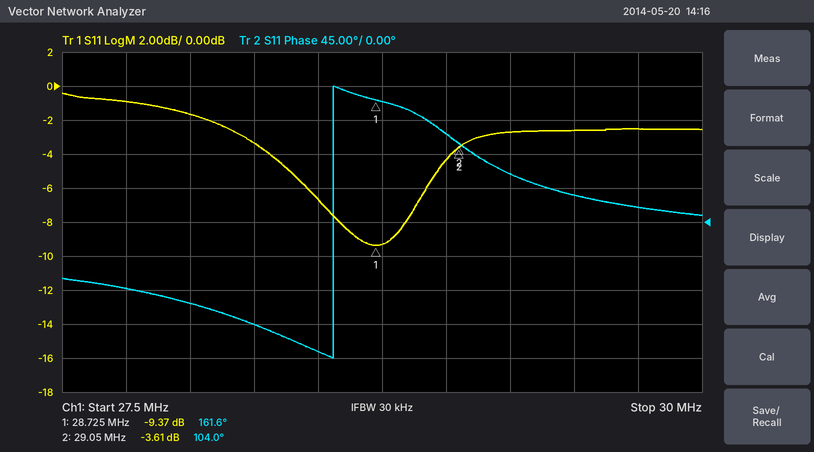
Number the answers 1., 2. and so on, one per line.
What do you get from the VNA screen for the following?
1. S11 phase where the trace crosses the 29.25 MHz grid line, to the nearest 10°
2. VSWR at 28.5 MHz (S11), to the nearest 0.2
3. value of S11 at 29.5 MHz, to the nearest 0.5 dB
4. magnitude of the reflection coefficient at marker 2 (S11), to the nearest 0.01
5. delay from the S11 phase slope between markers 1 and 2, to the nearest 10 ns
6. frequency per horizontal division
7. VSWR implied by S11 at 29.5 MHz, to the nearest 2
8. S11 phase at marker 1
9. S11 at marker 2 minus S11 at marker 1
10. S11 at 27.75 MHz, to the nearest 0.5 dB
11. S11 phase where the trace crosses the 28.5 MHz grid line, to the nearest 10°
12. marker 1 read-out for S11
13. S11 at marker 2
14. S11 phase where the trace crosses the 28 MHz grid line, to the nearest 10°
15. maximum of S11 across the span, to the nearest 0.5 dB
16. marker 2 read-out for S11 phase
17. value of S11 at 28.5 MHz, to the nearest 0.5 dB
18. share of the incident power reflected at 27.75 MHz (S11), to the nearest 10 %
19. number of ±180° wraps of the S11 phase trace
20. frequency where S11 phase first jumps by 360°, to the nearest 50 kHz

1. 60°
2. 2.8
3. -2.5 dB
4. 0.66
5. 490 ns
6. 250 kHz
7. 6
8. 161.6°
9. 5.76 dB
10. -1.0 dB
11. -170°
12. -9.37 dB
13. -3.61 dB
14. -110°
15. -0.5 dB
16. 104.0°
17. -6.5 dB
18. 80 %
19. 1
20. 28.55 MHz
